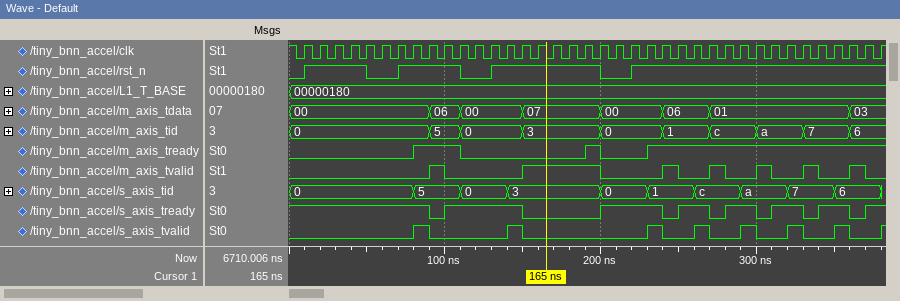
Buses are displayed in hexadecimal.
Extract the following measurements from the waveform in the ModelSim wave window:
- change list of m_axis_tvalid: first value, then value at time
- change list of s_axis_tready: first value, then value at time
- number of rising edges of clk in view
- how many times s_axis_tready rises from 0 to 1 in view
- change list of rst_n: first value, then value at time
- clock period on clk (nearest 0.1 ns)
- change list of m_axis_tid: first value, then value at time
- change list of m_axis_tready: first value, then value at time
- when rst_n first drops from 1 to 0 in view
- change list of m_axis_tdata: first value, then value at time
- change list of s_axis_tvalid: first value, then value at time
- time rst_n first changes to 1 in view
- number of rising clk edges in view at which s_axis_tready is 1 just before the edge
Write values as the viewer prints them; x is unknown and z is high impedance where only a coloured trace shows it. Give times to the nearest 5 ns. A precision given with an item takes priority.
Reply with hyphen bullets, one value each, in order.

- 0, 1 at 90 ns, 0 at 100 ns, 1 at 150 ns, 0 at 200 ns, 1 at 240 ns, 0 at 250 ns, 1 at 270 ns, 0 at 280 ns, 1 at 300 ns, 0 at 310 ns, 1 at 330 ns, 0 at 340 ns, 1 at 360 ns, 0 at 370 ns
- 1, 0 at 90 ns, 1 at 100 ns, 0 at 150 ns, 1 at 200 ns, 0 at 240 ns, 1 at 250 ns, 0 at 270 ns, 1 at 280 ns, 0 at 300 ns, 1 at 310 ns, 0 at 330 ns, 1 at 340 ns, 0 at 360 ns, 1 at 370 ns
- 38
- 7
- 0, 1 at 10 ns, 0 at 50 ns, 1 at 70 ns, 0 at 110 ns, 1 at 130 ns, 0 at 200 ns, 1 at 220 ns
- 10 ns
- 0, 5 at 90 ns, 0 at 110 ns, 3 at 150 ns, 0 at 200 ns, 1 at 240 ns, c at 270 ns, a at 300 ns, 7 at 330 ns, 6 at 360 ns
- 0, 1 at 80 ns, 0 at 110 ns, 1 at 190 ns, 0 at 200 ns, 1 at 230 ns
- 50 ns
- 00, 06 at 90 ns, 00 at 110 ns, 07 at 150 ns, 00 at 200 ns, 06 at 240 ns, 01 at 270 ns, 03 at 360 ns
- 0, 1 at 80 ns, 0 at 90 ns, 1 at 140 ns, 0 at 150 ns, 1 at 230 ns, 0 at 240 ns, 1 at 260 ns, 0 at 270 ns, 1 at 290 ns, 0 at 300 ns, 1 at 320 ns, 0 at 330 ns, 1 at 350 ns, 0 at 360 ns, 1 at 380 ns
- 10 ns
- 27
